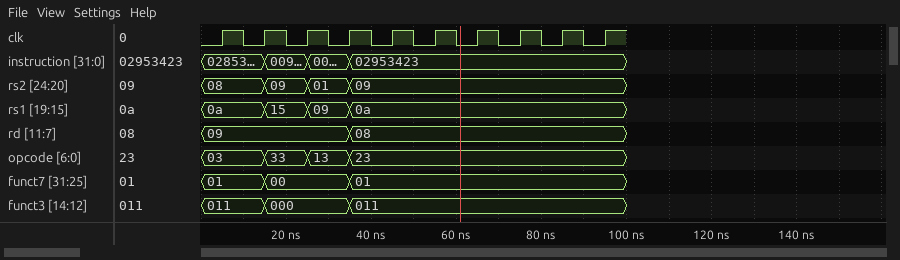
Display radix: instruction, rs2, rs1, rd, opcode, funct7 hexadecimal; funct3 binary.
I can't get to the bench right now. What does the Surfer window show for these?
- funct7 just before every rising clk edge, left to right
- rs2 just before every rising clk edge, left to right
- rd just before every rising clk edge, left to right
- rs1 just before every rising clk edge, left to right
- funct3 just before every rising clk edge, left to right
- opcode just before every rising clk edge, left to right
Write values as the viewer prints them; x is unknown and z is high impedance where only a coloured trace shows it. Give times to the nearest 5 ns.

01, 01, 00, 00, 01, 01, 01, 01, 01, 01
08, 08, 09, 01, 09, 09, 09, 09, 09, 09
09, 09, 09, 09, 08, 08, 08, 08, 08, 08
0a, 0a, 15, 09, 0a, 0a, 0a, 0a, 0a, 0a
011, 011, 000, 000, 011, 011, 011, 011, 011, 011
03, 03, 33, 13, 23, 23, 23, 23, 23, 23
